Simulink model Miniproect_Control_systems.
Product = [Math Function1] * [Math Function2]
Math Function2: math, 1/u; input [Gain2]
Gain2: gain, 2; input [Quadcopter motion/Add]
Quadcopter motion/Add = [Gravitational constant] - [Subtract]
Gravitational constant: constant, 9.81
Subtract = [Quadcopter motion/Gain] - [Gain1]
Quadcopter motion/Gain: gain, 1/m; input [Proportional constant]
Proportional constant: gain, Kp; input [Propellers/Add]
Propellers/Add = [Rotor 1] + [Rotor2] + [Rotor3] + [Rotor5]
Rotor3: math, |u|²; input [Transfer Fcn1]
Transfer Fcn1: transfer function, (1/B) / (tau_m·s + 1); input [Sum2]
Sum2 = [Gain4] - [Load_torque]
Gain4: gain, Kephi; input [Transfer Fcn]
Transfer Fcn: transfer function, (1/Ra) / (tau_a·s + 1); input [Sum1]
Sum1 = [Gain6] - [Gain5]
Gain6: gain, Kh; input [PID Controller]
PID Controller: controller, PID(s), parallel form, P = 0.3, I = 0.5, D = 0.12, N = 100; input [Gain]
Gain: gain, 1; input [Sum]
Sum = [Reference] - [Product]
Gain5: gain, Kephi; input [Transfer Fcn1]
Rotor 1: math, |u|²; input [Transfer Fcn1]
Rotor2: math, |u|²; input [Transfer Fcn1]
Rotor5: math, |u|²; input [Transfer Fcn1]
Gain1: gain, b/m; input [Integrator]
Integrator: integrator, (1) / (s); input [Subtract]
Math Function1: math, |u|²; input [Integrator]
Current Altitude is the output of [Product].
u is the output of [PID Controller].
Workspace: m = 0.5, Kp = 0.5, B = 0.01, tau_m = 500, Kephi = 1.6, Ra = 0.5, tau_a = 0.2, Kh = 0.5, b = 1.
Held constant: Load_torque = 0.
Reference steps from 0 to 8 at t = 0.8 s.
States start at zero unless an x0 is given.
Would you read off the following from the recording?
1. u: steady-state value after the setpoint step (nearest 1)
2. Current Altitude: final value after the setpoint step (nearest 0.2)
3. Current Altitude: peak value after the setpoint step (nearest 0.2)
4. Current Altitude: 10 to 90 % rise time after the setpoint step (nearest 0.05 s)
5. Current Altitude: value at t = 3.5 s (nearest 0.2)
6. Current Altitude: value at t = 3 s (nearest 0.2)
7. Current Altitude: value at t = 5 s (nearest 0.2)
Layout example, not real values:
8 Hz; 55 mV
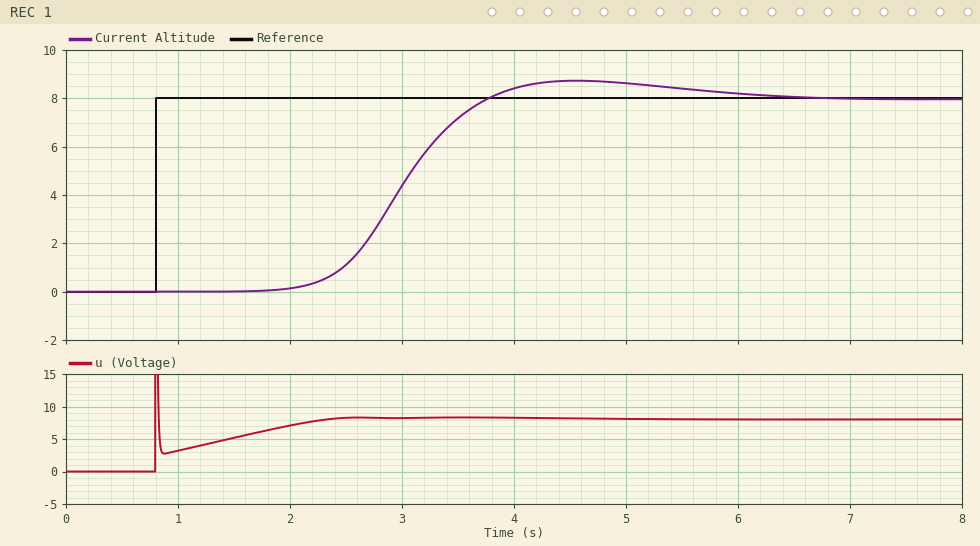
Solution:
8; 8.0; 8.8; 1.10 s; 7.2; 4.4; 8.6
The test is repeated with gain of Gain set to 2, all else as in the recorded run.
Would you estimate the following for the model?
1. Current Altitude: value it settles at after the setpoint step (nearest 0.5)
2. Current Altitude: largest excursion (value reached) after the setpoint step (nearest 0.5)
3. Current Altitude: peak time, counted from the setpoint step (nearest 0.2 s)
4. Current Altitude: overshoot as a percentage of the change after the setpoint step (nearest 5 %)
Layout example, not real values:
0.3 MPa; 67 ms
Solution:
8.0; 9.0; 2.4 s; 10 %
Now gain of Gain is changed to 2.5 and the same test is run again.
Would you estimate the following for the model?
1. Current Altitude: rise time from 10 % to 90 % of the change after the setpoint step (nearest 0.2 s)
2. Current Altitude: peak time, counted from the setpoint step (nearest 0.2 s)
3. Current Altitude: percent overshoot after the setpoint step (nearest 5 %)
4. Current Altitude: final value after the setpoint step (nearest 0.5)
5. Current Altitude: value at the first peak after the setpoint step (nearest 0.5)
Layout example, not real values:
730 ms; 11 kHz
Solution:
0.6 s; 2.2 s; 10 %; 8.0; 9.0
